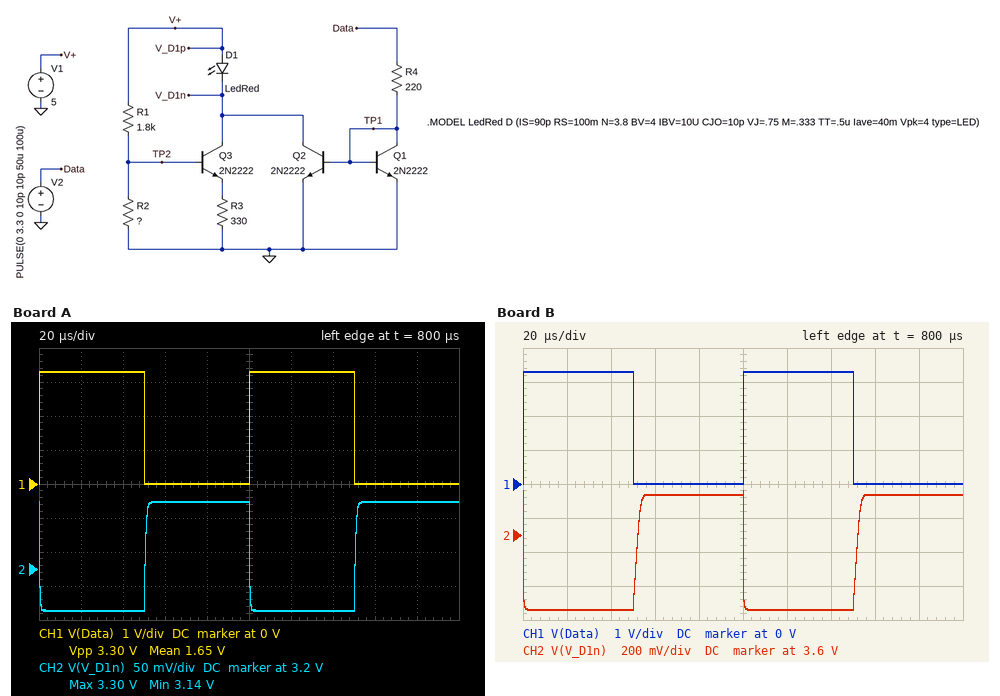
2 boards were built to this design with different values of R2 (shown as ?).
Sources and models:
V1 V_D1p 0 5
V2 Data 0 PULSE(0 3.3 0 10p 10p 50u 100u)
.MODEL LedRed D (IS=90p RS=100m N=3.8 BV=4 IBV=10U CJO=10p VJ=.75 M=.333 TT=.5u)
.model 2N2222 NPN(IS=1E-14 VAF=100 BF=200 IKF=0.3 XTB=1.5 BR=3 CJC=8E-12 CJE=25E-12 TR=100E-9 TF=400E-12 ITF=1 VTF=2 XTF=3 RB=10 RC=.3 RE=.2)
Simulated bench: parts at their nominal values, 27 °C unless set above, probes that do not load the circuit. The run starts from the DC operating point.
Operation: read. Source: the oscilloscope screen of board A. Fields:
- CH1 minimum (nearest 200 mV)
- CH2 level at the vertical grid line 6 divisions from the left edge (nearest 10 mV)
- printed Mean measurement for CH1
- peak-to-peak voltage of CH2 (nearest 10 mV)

0 V
3.14 V
1.65 V
160 mV
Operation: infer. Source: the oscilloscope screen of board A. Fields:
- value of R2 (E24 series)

910 Ω
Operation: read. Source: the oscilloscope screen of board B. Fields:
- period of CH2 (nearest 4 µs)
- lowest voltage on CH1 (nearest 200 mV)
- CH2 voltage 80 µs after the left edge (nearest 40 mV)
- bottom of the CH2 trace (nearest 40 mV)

100 µs
0 V
3.84 V
3.16 V
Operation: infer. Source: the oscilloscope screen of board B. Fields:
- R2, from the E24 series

220 Ω
